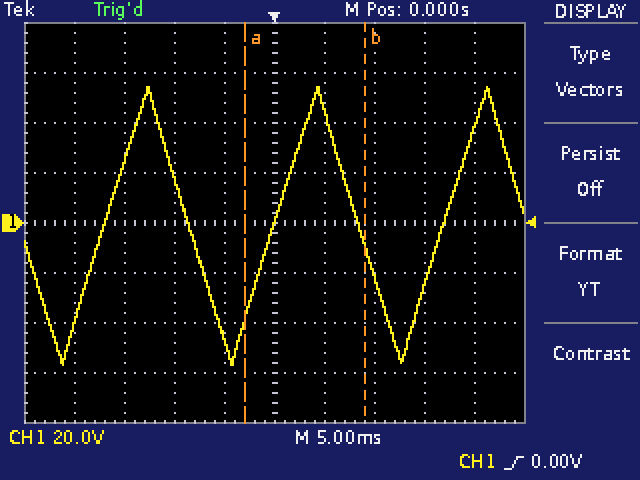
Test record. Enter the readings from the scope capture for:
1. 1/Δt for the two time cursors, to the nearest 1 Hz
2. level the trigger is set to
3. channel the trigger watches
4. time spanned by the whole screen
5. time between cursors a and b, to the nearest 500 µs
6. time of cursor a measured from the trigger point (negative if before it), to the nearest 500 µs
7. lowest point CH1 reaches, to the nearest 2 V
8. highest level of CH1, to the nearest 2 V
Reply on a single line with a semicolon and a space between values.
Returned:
83 Hz; 0.00 V; CH1; 50 ms; 12.0 ms; -3.0 ms; -56 V; 54 V
